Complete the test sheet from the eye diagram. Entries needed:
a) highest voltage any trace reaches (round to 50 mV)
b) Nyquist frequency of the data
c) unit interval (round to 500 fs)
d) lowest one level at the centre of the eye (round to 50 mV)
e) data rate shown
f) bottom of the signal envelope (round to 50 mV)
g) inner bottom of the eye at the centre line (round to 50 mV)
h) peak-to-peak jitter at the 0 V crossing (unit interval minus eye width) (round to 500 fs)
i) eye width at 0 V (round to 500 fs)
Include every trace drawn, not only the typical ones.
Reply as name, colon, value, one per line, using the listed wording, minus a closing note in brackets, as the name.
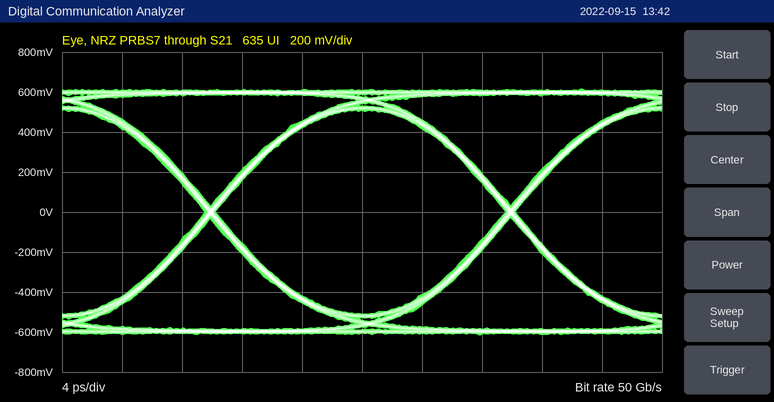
highest voltage any trace reaches: 600 mV
Nyquist frequency of the data: 25 GHz
unit interval: 20.0 ps
lowest one level at the centre of the eye: 500 mV
data rate shown: 50 Gb/s
bottom of the signal envelope: -600 mV
inner bottom of the eye at the centre line: -500 mV
peak-to-peak jitter at the 0 V crossing (unit interval minus eye width): 500 fs
eye width at 0 V: 19.5 ps
